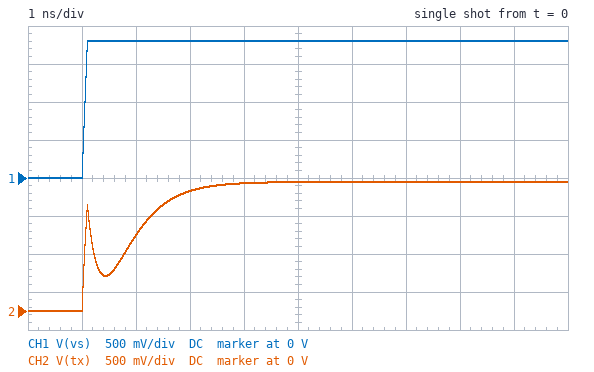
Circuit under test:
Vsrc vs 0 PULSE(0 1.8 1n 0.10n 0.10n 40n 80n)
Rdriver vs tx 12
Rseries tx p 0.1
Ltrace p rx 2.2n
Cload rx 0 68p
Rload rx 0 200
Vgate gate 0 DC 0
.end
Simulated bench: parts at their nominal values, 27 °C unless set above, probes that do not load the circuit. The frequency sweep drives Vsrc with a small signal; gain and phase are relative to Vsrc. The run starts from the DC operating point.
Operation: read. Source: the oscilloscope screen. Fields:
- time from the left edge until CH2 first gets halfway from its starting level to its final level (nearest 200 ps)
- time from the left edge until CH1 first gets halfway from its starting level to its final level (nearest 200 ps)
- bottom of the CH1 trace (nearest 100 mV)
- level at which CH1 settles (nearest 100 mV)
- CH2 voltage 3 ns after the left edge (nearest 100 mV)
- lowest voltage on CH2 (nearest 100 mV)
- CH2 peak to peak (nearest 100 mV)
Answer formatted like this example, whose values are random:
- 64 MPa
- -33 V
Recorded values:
- 1.0 ns
- 1.0 ns
- 0 V
- 1.8 V
- 1.6 V
- 0 V
- 1.7 V
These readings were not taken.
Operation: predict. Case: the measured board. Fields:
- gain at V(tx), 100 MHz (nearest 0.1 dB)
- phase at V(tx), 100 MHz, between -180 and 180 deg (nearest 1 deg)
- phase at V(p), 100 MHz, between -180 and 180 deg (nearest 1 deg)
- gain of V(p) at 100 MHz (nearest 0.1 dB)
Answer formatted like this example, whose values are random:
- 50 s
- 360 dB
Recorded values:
- -1.6 dB
- -27 deg
- -27 deg
- -1.6 dB
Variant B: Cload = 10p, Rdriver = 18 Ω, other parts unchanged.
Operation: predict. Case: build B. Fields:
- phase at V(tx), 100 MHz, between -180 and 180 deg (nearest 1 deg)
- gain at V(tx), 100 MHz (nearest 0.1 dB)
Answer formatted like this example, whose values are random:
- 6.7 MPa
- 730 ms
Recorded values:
- -6 deg
- -0.8 dB
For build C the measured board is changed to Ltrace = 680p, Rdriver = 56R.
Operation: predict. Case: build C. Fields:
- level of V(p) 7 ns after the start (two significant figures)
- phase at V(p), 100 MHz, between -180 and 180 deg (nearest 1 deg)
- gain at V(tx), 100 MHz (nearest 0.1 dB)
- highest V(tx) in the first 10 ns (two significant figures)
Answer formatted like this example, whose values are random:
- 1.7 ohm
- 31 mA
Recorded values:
- 1.2 V
- -62 deg
- -8.8 dB
- 1.3 V
